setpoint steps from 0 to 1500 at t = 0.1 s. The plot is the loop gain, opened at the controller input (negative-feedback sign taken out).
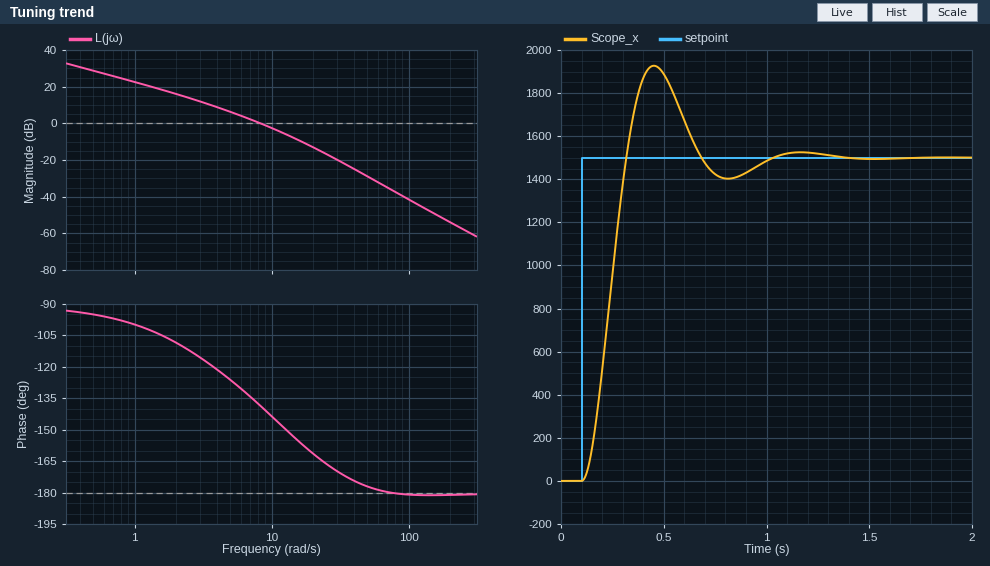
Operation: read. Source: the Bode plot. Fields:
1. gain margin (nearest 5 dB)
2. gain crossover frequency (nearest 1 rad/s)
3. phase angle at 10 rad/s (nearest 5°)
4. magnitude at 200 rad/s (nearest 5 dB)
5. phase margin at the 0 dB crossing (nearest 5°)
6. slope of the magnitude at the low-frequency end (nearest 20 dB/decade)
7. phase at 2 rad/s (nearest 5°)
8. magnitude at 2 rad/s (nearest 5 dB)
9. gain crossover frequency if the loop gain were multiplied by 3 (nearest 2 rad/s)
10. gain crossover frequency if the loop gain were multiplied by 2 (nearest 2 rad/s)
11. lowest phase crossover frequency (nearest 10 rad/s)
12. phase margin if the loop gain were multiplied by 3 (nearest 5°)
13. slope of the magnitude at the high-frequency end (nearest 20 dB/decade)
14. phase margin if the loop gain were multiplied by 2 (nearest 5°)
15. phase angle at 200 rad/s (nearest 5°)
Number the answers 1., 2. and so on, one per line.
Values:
1. 35 dB
2. 8 rad/s
3. -145°
4. -55 dB
5. 40°
6. -20 dB/decade
7. -110°
8. 15 dB
9. 16 rad/s
10. 12 rad/s
11. 70 rad/s
12. 25°
13. -40 dB/decade
14. 30°
15. -180°
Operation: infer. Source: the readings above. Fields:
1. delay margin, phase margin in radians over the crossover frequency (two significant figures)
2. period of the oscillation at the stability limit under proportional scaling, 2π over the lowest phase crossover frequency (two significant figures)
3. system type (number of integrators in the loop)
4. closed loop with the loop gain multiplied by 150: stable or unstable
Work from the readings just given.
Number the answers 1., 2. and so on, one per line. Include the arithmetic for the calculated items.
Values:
1. 40 × π / 180 / 8 = 0.087 s
2. 2π / 70 = 0.090 s
3. 1
4. unstable
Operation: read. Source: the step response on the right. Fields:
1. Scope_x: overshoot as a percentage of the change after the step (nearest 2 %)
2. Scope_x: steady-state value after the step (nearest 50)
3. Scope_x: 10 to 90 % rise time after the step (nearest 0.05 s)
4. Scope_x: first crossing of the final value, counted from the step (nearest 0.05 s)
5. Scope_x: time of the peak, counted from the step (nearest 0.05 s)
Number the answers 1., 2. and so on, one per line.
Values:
1. 28 %
2. 1500
3. 0.15 s
4. 0.20 s
5. 0.35 s
